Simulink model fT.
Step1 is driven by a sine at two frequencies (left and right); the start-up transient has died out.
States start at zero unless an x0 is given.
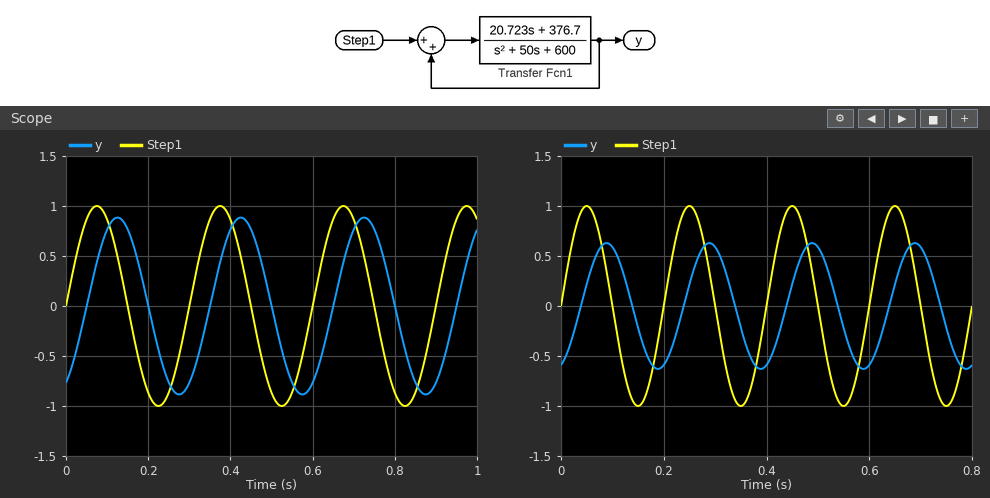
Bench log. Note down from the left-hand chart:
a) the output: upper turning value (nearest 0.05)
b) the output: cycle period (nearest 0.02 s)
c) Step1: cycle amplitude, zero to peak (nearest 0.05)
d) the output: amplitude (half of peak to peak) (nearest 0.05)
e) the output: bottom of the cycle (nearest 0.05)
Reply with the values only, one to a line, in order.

0.90
0.30 s
1.00
0.90
-0.90
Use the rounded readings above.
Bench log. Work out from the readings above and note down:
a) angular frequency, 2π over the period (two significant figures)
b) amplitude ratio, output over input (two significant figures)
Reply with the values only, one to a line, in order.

21 rad/s
0.90
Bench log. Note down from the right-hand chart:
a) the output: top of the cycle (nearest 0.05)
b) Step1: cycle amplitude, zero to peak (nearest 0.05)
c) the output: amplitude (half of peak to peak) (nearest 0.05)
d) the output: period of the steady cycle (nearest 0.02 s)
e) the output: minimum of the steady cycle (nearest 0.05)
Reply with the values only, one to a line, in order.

0.65
1.00
0.65
0.20 s
-0.65
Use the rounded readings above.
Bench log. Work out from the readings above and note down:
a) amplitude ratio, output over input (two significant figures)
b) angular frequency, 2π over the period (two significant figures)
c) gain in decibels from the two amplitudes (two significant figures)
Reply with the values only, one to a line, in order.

0.65
31 rad/s
-3.7 dB
